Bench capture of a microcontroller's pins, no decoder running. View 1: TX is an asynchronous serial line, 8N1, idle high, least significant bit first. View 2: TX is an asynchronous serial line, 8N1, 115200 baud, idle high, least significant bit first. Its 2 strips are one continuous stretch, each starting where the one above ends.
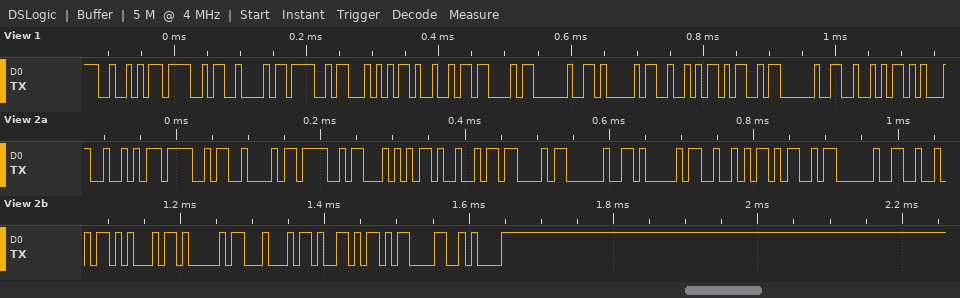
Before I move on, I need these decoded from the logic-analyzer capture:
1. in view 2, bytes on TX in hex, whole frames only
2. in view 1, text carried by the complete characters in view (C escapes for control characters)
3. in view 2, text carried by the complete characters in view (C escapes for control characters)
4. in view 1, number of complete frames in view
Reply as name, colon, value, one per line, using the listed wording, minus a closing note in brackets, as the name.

in view 2, bytes on TX in hex, whole frames only: 52 4F 42 4F 54 49 43 20 41 52 4D 20 52 45 41 44 59 0D 0A
in view 1, text carried by the complete characters in view: "ROBOTIC ARM R"
in view 2, text carried by the complete characters in view: "ROBOTIC ARM READY\r\n"
in view 1, number of complete frames in view: 13
